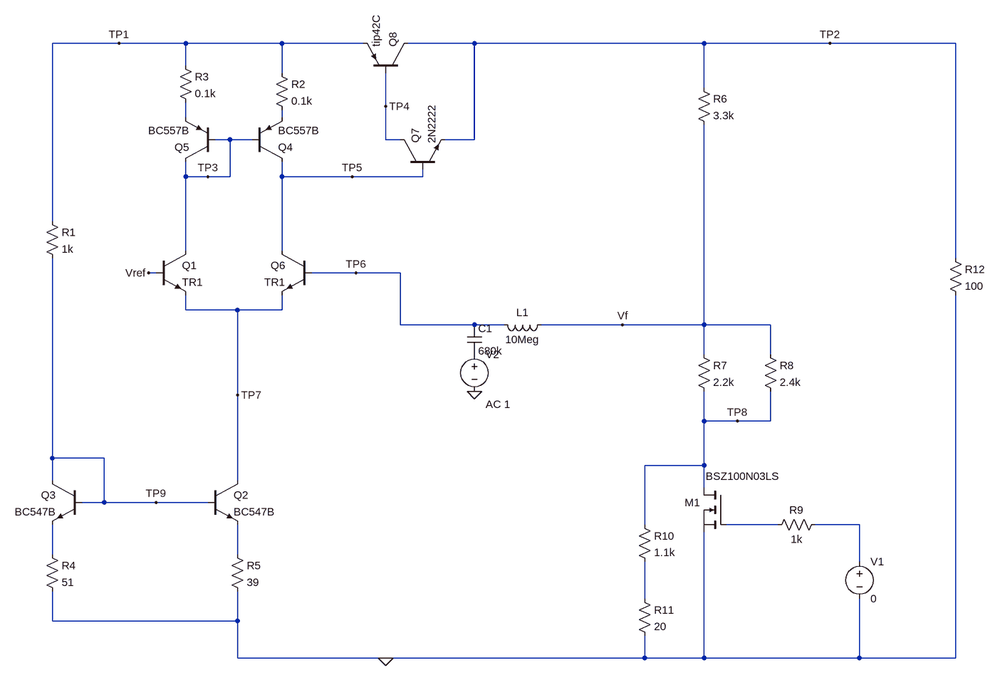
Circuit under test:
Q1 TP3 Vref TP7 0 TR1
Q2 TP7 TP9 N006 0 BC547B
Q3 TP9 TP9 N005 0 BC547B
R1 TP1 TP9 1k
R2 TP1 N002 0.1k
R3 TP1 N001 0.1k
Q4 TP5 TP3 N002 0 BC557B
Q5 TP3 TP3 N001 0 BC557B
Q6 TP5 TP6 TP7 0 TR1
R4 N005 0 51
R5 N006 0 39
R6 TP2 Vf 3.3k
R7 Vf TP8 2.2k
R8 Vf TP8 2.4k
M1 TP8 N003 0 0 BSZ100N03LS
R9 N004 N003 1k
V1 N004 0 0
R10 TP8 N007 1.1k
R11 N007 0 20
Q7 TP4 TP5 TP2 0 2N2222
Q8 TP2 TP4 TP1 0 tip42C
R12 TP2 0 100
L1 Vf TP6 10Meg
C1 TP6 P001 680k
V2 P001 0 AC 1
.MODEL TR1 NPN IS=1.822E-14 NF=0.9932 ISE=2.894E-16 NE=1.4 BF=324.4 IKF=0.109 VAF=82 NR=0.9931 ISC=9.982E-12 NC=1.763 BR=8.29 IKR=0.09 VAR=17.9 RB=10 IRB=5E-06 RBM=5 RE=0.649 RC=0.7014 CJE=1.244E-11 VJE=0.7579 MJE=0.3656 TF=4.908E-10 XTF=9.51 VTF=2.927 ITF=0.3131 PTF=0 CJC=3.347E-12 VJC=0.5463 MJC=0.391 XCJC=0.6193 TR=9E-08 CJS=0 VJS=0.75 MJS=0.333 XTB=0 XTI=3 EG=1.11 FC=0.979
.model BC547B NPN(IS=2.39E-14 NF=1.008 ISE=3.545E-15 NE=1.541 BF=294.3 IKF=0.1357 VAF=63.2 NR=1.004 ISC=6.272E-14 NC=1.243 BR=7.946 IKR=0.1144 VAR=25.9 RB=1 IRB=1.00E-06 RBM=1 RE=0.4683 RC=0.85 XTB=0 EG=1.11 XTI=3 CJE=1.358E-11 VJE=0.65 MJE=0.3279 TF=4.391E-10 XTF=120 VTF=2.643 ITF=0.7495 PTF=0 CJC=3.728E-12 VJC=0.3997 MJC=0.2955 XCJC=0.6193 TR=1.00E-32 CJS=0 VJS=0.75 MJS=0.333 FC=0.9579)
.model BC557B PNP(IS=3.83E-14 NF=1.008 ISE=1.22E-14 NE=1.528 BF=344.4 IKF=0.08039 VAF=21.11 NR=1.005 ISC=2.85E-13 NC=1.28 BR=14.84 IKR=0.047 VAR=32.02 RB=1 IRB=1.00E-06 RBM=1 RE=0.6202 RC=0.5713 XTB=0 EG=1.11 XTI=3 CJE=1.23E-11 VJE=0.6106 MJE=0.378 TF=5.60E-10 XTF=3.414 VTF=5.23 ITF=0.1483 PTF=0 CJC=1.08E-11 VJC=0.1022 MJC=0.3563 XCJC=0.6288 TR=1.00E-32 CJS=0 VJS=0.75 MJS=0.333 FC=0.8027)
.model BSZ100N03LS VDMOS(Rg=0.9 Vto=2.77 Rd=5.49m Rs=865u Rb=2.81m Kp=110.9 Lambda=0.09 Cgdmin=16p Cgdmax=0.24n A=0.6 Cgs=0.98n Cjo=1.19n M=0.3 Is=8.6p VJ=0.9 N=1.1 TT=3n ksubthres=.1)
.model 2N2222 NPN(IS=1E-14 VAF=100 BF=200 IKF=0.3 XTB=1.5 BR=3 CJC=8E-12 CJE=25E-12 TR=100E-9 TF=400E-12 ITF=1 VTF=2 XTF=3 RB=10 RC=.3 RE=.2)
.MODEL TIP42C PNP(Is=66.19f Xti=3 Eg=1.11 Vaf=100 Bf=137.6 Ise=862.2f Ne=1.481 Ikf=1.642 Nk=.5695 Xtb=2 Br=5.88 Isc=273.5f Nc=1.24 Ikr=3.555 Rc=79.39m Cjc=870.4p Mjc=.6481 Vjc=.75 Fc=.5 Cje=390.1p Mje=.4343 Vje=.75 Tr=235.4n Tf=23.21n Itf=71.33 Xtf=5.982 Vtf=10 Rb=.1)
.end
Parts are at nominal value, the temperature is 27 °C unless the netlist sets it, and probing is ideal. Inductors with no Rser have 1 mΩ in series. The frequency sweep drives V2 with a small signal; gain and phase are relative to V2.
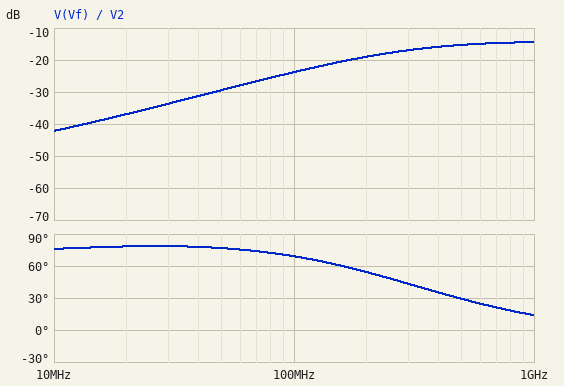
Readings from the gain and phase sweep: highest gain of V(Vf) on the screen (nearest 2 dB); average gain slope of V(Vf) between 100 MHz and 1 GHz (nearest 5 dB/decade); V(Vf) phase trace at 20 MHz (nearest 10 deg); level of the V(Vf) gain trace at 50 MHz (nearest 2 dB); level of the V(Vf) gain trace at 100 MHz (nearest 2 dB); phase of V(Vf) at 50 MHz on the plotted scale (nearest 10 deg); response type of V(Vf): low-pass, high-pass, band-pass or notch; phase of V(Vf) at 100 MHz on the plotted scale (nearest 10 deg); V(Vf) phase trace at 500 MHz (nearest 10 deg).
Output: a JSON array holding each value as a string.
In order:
["-14 dB", "10 dB/decade", "80 deg", "-30 dB", "-24 dB", "80 deg", "high-pass", "70 deg", "30 deg"]
